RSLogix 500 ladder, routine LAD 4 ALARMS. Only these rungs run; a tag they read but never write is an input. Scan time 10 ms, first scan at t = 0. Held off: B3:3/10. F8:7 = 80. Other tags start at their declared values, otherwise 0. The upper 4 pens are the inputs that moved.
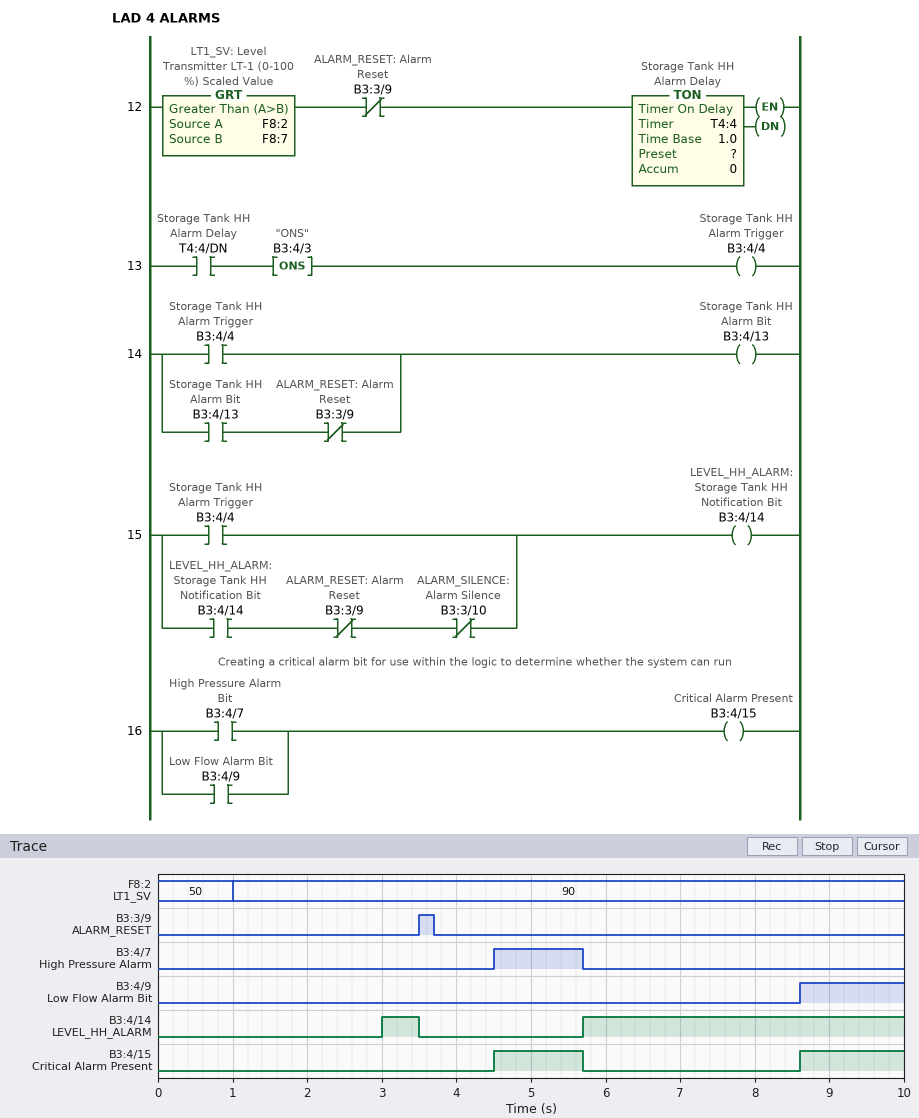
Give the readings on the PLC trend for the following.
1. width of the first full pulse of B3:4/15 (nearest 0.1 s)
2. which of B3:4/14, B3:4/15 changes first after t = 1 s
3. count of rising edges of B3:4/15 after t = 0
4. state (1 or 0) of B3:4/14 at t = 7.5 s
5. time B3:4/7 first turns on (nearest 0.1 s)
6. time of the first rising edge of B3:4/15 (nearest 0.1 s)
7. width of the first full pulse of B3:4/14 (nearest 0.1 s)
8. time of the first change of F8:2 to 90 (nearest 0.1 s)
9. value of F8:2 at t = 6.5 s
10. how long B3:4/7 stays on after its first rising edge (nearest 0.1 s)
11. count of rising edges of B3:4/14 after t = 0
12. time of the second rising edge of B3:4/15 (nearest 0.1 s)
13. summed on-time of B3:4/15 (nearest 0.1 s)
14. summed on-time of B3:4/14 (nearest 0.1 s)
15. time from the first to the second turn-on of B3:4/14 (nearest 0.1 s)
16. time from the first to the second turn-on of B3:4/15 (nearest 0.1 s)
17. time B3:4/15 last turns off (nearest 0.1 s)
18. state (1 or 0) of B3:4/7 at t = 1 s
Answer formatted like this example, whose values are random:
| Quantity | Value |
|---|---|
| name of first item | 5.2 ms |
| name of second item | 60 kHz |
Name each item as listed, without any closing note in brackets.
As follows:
| Quantity | Value |
|---|---|
| width of the first full pulse of B3:4/15 | 1.2 s |
| which of B3:4/14, B3:4/15 changes first after t = 1 s | B3:4/14 |
| count of rising edges of B3:4/15 after t = 0 | 2 |
| state (1 or 0) of B3:4/14 at t = 7.5 s | 1 |
| time B3:4/7 first turns on | 4.5 s |
| time of the first rising edge of B3:4/15 | 4.5 s |
| width of the first full pulse of B3:4/14 | 0.5 s |
| time of the first change of F8:2 to 90 | 1.0 s |
| value of F8:2 at t = 6.5 s | 90 |
| how long B3:4/7 stays on after its first rising edge | 1.2 s |
| count of rising edges of B3:4/14 after t = 0 | 2 |
| time of the second rising edge of B3:4/15 | 8.6 s |
| summed on-time of B3:4/15 | 2.6 s |
| summed on-time of B3:4/14 | 4.8 s |
| time from the first to the second turn-on of B3:4/14 | 2.7 s |
| time from the first to the second turn-on of B3:4/15 | 4.1 s |
| time B3:4/15 last turns off | 5.7 s |
| state (1 or 0) of B3:4/7 at t = 1 s | 0 |
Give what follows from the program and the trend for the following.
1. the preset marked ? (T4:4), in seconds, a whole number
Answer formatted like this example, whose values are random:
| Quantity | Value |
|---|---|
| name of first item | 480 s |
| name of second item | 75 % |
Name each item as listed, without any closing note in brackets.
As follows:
| Quantity | Value |
|---|---|
| the preset marked ? (T4:4), in seconds, a whole number | 2 s |
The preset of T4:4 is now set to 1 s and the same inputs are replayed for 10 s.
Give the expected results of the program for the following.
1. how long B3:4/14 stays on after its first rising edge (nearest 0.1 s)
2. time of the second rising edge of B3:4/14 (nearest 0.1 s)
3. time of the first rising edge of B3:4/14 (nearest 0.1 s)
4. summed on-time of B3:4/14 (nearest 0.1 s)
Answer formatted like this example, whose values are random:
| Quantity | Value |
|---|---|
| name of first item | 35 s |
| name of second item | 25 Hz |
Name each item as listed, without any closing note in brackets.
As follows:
| Quantity | Value |
|---|---|
| how long B3:4/14 stays on after its first rising edge | 1.5 s |
| time of the second rising edge of B3:4/14 | 4.7 s |
| time of the first rising edge of B3:4/14 | 2.0 s |
| summed on-time of B3:4/14 | 6.8 s |
